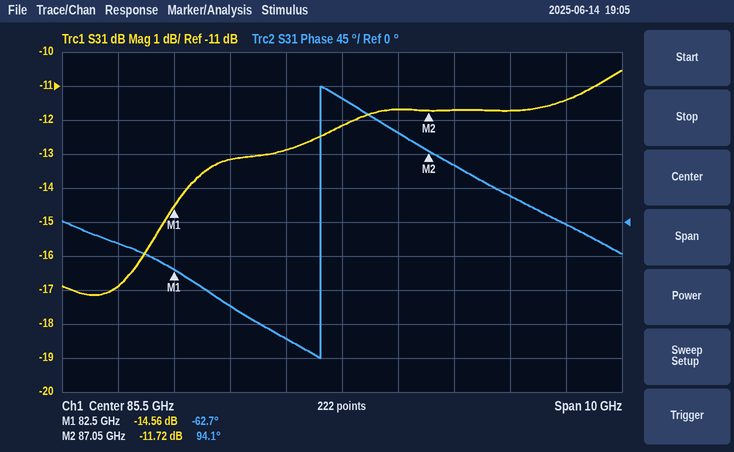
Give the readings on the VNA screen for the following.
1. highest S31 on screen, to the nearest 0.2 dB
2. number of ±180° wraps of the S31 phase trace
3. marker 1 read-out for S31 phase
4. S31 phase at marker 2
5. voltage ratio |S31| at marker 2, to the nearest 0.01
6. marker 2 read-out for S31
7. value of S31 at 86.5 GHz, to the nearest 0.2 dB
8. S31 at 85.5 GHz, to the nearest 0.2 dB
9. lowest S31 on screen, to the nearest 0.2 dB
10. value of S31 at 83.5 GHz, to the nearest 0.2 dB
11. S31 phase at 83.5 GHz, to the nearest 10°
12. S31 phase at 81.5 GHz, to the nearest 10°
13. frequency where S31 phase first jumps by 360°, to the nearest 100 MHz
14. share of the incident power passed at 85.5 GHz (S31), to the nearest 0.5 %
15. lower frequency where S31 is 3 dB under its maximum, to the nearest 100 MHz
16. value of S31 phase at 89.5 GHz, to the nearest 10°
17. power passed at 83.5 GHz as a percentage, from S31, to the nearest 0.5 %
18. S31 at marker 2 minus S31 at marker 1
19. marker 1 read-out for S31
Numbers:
-10.6 dB
1
-62.7°
94.1°
0.26
-11.72 dB
-11.6 dB
-12.2 dB
-17.2 dB
-13.2 dB
-110°
-30°
85.1 GHz
6.0 %
83.0 GHz
0°
5.0 %
2.84 dB
-14.56 dB
